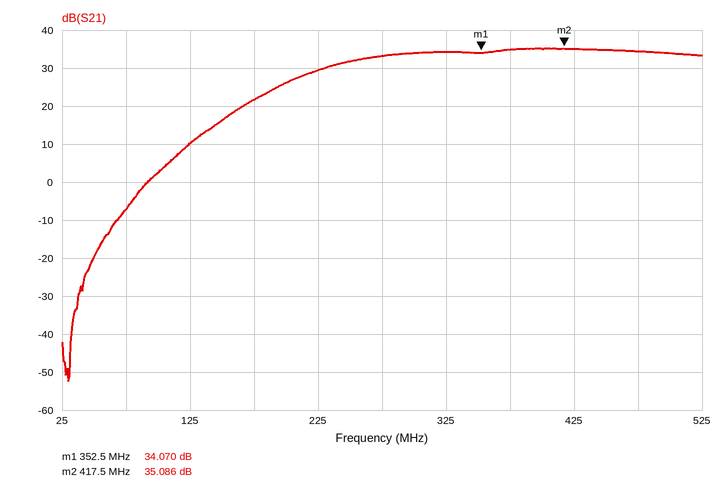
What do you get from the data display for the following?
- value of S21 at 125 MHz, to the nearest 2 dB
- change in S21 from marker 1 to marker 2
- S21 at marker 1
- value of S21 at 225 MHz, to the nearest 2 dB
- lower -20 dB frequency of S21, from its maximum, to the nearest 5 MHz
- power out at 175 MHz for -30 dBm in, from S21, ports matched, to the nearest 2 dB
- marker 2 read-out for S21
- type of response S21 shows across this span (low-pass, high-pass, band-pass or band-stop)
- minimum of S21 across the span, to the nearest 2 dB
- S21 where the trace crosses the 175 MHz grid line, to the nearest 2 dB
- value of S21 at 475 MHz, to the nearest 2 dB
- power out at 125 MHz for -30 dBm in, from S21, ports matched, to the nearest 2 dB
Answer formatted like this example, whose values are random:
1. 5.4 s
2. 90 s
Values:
1. 10 dB
2. 1.016 dB
3. 34.070 dB
4. 30 dB
5. 145 MHz
6. -8 dBm
7. 35.086 dB
8. high-pass
9. -52 dB
10. 22 dB
11. 34 dB
12. -20 dBm
